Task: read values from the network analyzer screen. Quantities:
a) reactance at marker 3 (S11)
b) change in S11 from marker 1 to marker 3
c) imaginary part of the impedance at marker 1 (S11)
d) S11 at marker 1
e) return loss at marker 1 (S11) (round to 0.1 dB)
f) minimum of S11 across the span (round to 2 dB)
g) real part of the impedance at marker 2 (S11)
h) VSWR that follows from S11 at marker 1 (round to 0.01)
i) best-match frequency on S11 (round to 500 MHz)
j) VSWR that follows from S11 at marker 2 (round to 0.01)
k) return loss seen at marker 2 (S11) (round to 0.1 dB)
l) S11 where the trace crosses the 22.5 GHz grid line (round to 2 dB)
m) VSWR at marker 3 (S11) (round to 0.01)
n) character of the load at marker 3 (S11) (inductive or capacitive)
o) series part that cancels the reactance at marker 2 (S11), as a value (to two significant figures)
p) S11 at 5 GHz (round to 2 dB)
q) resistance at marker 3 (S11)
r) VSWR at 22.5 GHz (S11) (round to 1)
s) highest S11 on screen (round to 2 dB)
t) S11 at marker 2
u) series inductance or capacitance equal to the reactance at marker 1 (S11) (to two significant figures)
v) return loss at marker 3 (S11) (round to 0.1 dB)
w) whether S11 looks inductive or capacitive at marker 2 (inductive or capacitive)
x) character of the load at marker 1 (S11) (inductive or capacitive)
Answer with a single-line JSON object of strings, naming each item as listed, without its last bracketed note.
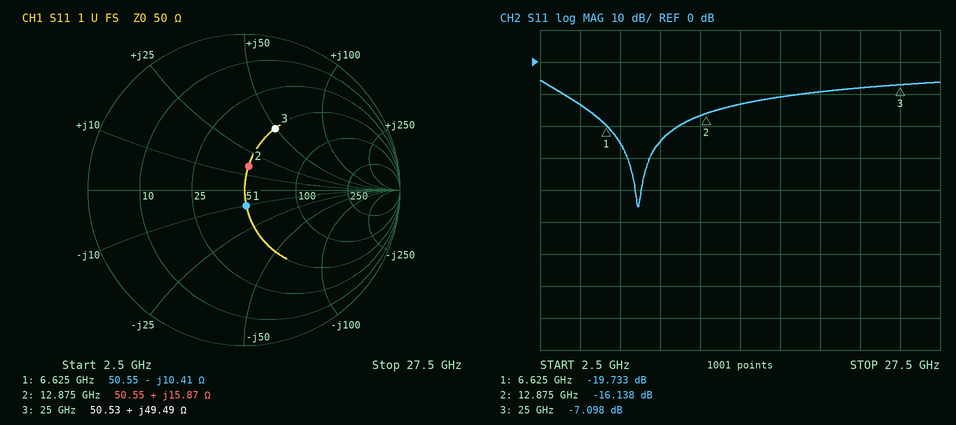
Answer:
{"reactance at marker 3": "+49.49 Ω", "change in S11 from marker 1 to marker 3": "12.635 dB", "imaginary part of the impedance at marker 1": "-10.41 Ω", "S11 at marker 1": "-19.733 dB", "return loss at marker 1 (S11)": "19.7 dB", "minimum of S11 across the span": "-46 dB", "real part of the impedance at marker 2": "50.55 Ω", "VSWR that follows from S11 at marker 1": "1.23", "best-match frequency on S11": "8.5 GHz", "VSWR that follows from S11 at marker 2": "1.37", "return loss seen at marker 2 (S11)": "16.1 dB", "S11 where the trace crosses the 22.5 GHz grid line": "-8 dB", "VSWR at marker 3 (S11)": "2.58", "character of the load at marker 3 (S11)": "inductive", "series part that cancels the reactance at marker 2 (S11), as a value": "780 fF", "S11 at 5 GHz": "-14 dB", "resistance at marker 3": "50.53 Ω", "VSWR at 22.5 GHz (S11)": "2", "highest S11 on screen": "-6 dB", "S11 at marker 2": "-16.138 dB", "series inductance or capacitance equal to the reactance at marker 1 (S11)": "2.3 pF", "return loss at marker 3 (S11)": "7.1 dB", "whether S11 looks inductive or capacitive at marker 2": "inductive", "character of the load at marker 1 (S11)": "capacitive"}
